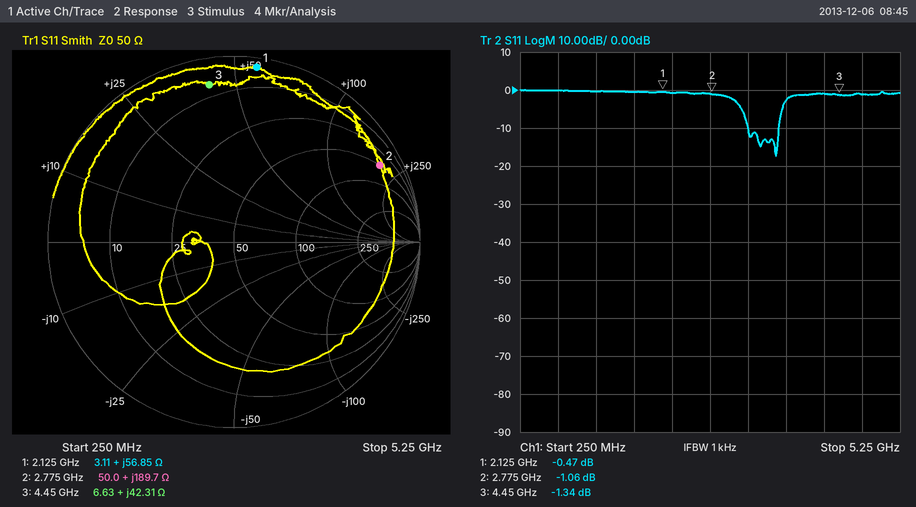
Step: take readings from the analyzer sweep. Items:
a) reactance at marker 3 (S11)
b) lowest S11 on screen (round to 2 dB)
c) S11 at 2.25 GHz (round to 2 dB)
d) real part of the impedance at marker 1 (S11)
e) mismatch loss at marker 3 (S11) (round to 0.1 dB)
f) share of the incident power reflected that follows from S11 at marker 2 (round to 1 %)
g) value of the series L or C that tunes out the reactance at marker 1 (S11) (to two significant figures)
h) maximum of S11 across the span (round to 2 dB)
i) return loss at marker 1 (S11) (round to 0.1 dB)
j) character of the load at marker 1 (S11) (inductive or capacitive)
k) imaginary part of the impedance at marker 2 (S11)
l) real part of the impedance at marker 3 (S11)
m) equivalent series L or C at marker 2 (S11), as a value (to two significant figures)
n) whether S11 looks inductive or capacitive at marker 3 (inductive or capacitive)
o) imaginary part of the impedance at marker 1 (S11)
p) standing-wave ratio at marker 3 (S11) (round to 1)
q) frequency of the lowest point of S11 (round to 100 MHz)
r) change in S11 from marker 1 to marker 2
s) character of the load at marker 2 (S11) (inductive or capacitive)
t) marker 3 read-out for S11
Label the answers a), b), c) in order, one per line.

a) +42.31 Ω
b) -18 dB
c) 0 dB
d) 3.11 Ω
e) 5.8 dB
f) 78 %
g) 1.3 pF
h) 0 dB
i) 0.5 dB
j) inductive
k) +189.7 Ω
l) 6.63 Ω
m) 11 nH
n) inductive
o) +56.85 Ω
p) 13
q) 3.6 GHz
r) -0.59 dB
s) inductive
t) -1.34 dB
